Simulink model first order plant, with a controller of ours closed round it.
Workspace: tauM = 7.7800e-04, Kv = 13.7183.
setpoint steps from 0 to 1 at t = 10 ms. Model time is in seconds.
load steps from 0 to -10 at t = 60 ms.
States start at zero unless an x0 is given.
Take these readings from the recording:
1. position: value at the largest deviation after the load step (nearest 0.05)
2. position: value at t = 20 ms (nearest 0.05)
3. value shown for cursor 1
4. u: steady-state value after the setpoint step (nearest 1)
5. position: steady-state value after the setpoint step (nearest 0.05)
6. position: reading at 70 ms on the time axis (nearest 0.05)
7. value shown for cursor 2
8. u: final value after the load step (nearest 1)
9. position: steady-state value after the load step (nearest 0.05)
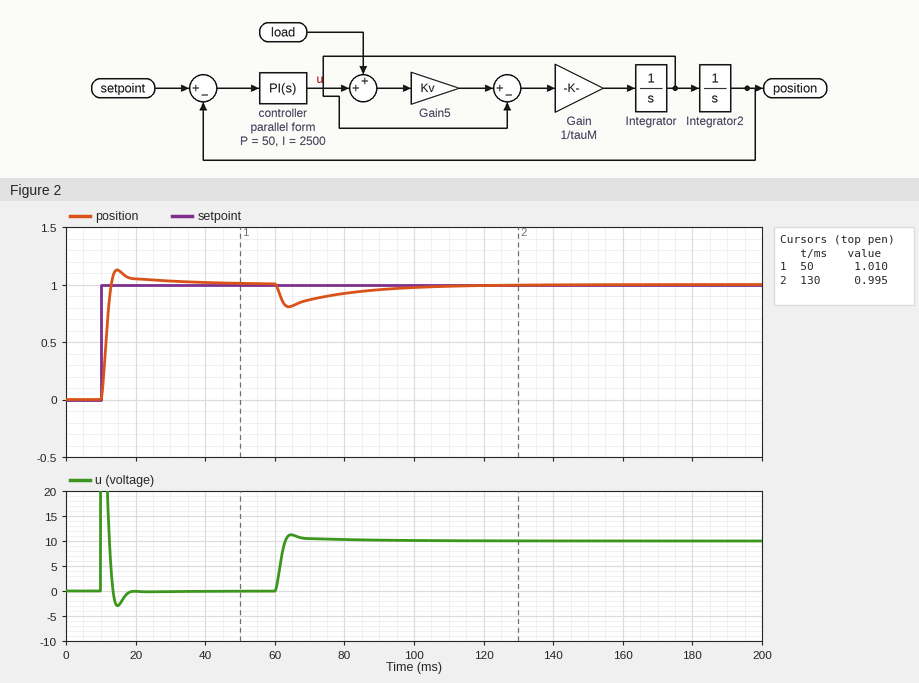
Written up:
0.80
1.05
1.010
0
1.00
0.85
0.995
10
1.00
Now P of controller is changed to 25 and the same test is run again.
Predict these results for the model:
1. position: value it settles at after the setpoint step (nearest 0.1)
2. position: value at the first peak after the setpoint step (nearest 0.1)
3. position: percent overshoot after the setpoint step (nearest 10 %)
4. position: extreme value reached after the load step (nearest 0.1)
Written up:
1.0
1.2
20 %
0.7
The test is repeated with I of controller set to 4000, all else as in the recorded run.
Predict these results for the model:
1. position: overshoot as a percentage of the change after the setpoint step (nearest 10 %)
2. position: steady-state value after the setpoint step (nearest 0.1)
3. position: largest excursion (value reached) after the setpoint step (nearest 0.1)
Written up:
20 %
1.0
1.2
